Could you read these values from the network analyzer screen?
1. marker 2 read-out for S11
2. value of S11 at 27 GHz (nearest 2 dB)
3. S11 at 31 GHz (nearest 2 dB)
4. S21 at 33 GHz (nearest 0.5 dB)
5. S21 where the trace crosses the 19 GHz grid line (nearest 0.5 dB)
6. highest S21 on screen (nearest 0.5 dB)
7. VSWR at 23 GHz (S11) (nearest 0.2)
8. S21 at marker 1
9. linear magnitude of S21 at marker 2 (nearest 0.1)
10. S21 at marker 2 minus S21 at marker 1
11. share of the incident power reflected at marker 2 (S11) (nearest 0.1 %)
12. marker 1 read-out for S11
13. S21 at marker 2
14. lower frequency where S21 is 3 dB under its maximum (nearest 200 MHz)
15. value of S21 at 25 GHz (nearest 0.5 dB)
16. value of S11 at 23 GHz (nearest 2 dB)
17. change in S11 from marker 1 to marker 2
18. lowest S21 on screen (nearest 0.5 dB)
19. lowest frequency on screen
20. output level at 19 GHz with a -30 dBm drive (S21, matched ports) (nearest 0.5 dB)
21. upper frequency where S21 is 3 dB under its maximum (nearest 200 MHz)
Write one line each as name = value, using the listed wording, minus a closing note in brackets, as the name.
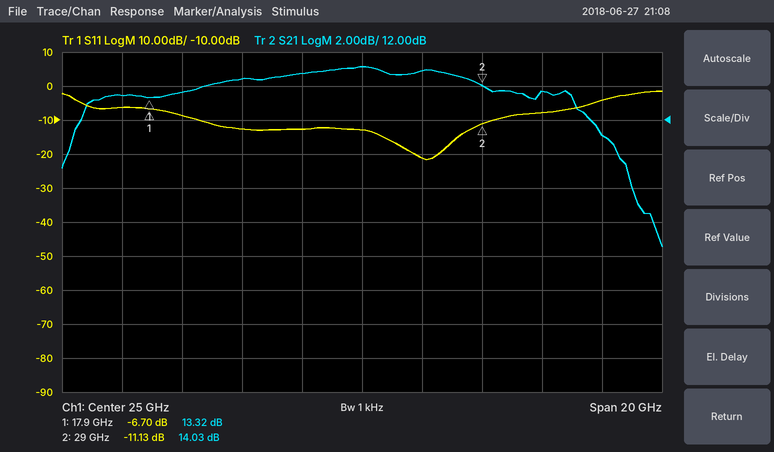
marker 2 read-out for S11 = -11.13 dB
value of S11 at 27 GHz = -22 dB
S11 at 31 GHz = -8 dB
S21 at 33 GHz = 11.0 dB
S21 where the trace crosses the 19 GHz grid line = 13.5 dB
highest S21 on screen = 15.0 dB
VSWR at 23 GHz (S11) = 1.6
S21 at marker 1 = 13.32 dB
linear magnitude of S21 at marker 2 = 5.0
S21 at marker 2 minus S21 at marker 1 = 0.71 dB
share of the incident power reflected at marker 2 (S11) = 7.7 %
marker 1 read-out for S11 = -6.70 dB
S21 at marker 2 = 14.03 dB
lower frequency where S21 is 3 dB under its maximum = 15.6 GHz
value of S21 at 25 GHz = 15.0 dB
value of S11 at 23 GHz = -12 dB
change in S11 from marker 1 to marker 2 = -4.43 dB
lowest S21 on screen = 4.5 dB
lowest frequency on screen = 15 GHz
output level at 19 GHz with a -30 dBm drive (S21, matched ports) = -16.5 dBm
upper frequency where S21 is 3 dB under its maximum = 32.6 GHz
